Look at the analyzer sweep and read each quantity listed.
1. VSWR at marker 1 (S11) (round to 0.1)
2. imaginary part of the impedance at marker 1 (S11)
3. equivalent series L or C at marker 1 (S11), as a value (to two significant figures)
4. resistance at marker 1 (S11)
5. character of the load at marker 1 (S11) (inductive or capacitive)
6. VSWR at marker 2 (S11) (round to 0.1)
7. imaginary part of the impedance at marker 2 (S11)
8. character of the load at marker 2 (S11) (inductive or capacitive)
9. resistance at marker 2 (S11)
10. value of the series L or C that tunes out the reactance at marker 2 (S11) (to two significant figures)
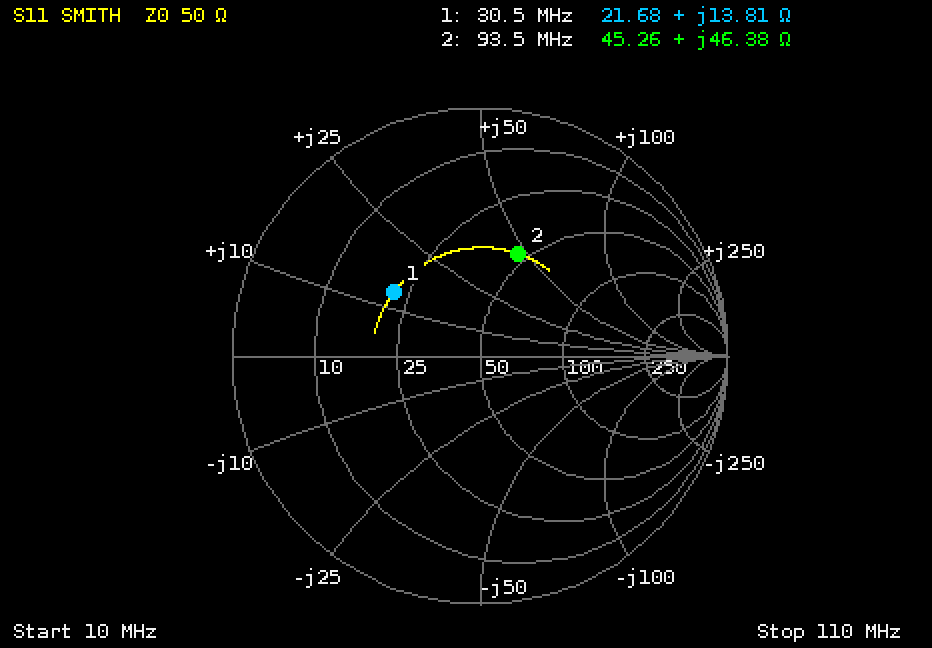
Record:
2.5
+13.81 Ω
72 nH
21.68 Ω
inductive
2.6
+46.38 Ω
inductive
45.26 Ω
37 pF
